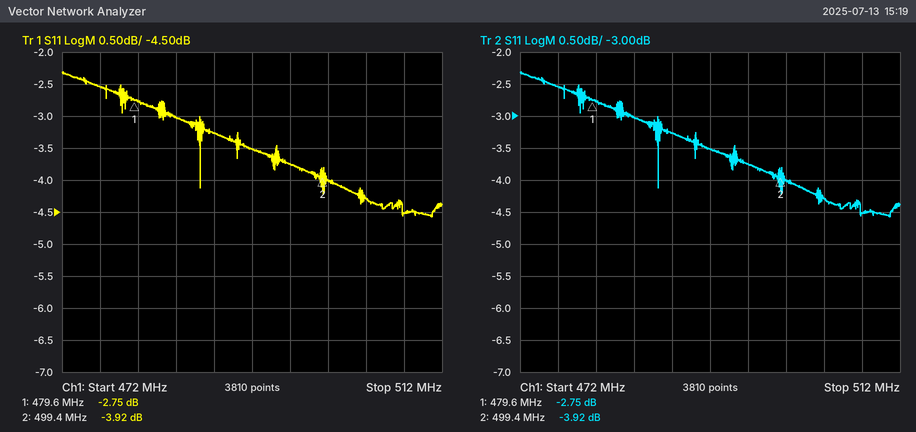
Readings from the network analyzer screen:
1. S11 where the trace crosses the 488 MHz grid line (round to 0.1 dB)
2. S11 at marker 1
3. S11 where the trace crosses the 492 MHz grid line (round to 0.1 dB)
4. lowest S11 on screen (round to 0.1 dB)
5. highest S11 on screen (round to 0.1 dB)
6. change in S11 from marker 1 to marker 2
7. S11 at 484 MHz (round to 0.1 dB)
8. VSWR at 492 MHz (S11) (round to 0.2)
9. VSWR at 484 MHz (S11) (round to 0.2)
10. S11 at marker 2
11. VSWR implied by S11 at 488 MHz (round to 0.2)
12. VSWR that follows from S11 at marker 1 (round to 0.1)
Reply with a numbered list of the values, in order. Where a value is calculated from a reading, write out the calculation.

1. -3.3 dB
2. -2.75 dB
3. -3.5 dB
4. -4.6 dB
5. -2.3 dB
6. -3.92 − (-2.75) = -1.17 dB
7. -3.0 dB
8. |Γ| = 10^(-3.5/20) = 0.6683; VSWR = (1 + 0.6683)/(1 − 0.6683) ≈ 5.0
9. |Γ| = 10^(-3/20) = 0.7079; VSWR = (1 + 0.7079)/(1 − 0.7079) ≈ 5.8
10. -3.92 dB
11. |Γ| = 10^(-3.3/20) = 0.6839; VSWR = (1 + 0.6839)/(1 − 0.6839) ≈ 5.33, so 5.4 to the nearest 0.2
12. (1 + 0.7286)/(1 − 0.7286) ≈ 6.4
